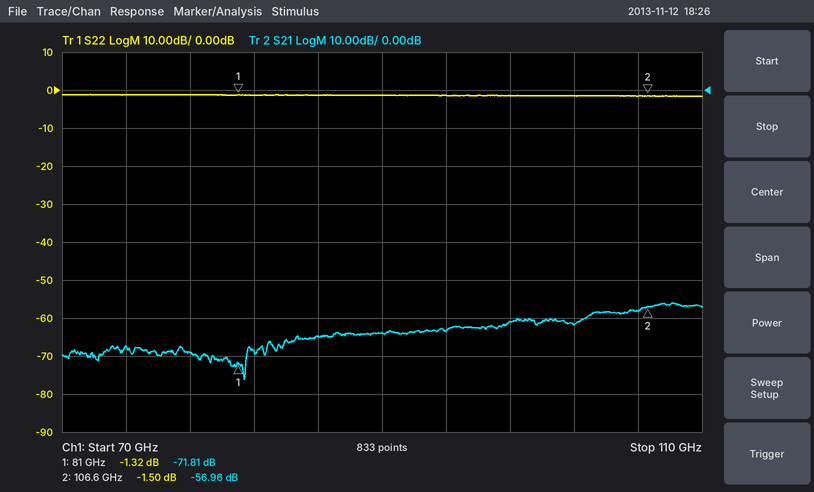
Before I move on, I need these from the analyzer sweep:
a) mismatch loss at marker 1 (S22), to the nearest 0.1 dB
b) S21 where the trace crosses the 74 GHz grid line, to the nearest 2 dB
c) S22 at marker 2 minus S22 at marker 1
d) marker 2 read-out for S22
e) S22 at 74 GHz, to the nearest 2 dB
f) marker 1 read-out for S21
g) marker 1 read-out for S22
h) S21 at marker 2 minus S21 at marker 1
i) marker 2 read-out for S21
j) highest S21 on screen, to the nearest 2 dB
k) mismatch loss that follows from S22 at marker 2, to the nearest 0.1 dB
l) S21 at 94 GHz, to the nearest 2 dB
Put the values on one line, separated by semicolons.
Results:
5.8 dB; -68 dB; -0.18 dB; -1.50 dB; -2 dB; -71.81 dB; -1.32 dB; 14.85 dB; -56.96 dB; -56 dB; 5.3 dB; -64 dB
